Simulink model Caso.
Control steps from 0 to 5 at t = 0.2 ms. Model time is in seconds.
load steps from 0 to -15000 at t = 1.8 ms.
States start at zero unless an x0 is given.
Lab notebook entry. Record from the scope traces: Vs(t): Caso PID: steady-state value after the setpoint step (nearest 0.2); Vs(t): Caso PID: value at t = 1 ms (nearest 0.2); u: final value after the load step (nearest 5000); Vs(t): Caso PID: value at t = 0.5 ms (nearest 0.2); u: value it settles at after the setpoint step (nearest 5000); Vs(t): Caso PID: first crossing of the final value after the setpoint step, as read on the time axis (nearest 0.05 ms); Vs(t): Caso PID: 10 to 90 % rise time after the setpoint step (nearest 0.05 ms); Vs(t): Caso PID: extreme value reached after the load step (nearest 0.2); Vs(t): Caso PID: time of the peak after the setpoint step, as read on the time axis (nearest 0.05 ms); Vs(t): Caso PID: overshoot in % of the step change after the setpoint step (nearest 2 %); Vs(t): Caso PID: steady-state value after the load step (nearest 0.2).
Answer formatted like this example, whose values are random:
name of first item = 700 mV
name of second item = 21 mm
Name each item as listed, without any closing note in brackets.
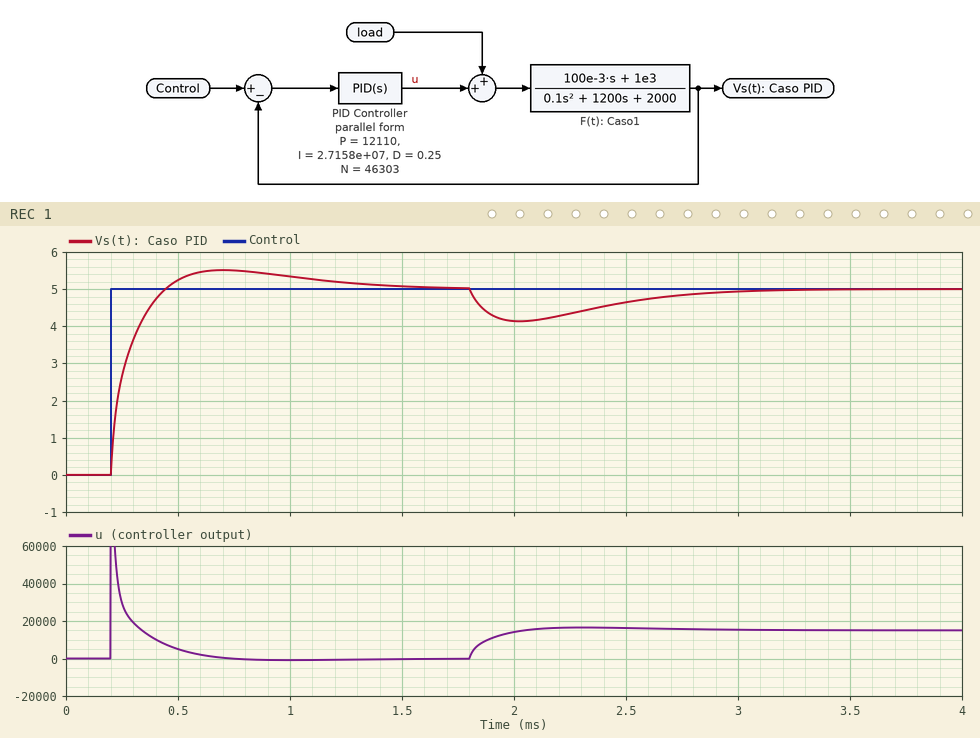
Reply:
Vs(t): Caso PID: steady-state value after the setpoint step = 5.0
Vs(t): Caso PID: value at t = 1 ms = 5.4
u: final value after the load step = 15000
Vs(t): Caso PID: value at t = 0.5 ms = 5.2
u: value it settles at after the setpoint step = 0
Vs(t): Caso PID: first crossing of the final value after the setpoint step, as read on the time axis = 0.45 ms
Vs(t): Caso PID: 10 to 90 % rise time after the setpoint step = 0.15 ms
Vs(t): Caso PID: extreme value reached after the load step = 4.2
Vs(t): Caso PID: time of the peak after the setpoint step, as read on the time axis = 0.70 ms
Vs(t): Caso PID: overshoot in % of the step change after the setpoint step = 10 %
Vs(t): Caso PID: steady-state value after the load step = 5.0
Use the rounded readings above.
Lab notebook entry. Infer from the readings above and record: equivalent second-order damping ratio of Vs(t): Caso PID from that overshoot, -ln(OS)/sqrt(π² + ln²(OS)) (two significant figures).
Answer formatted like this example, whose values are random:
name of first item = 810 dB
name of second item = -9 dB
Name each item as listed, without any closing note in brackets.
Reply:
equivalent second-order damping ratio of Vs(t): Caso PID from that overshoot, -ln(OS)/sqrt(π² + ln²(OS)) = 0.59
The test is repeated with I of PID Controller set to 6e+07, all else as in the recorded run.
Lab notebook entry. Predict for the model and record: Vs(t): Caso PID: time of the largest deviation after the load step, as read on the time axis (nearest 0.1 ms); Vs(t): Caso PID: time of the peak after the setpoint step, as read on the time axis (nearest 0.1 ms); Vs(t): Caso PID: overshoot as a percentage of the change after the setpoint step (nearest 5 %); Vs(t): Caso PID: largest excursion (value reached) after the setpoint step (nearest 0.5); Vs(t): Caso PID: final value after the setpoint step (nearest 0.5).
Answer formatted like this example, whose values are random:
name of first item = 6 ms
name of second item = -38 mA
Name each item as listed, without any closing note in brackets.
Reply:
Vs(t): Caso PID: time of the largest deviation after the load step, as read on the time axis = 2.0 ms
Vs(t): Caso PID: time of the peak after the setpoint step, as read on the time axis = 0.6 ms
Vs(t): Caso PID: overshoot as a percentage of the change after the setpoint step = 15 %
Vs(t): Caso PID: largest excursion (value reached) after the setpoint step = 6.0
Vs(t): Caso PID: final value after the setpoint step = 5.0
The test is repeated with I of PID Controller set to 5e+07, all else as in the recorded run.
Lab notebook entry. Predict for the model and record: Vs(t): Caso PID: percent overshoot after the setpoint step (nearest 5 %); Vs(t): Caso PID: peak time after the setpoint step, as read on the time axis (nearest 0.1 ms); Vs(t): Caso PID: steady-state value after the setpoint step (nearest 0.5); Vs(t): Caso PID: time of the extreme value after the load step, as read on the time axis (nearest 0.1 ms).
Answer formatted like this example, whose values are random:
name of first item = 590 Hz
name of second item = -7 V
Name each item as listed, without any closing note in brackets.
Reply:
Vs(t): Caso PID: percent overshoot after the setpoint step = 15 %
Vs(t): Caso PID: peak time after the setpoint step, as read on the time axis = 0.6 ms
Vs(t): Caso PID: steady-state value after the setpoint step = 5.0
Vs(t): Caso PID: time of the extreme value after the load step, as read on the time axis = 2.0 ms
